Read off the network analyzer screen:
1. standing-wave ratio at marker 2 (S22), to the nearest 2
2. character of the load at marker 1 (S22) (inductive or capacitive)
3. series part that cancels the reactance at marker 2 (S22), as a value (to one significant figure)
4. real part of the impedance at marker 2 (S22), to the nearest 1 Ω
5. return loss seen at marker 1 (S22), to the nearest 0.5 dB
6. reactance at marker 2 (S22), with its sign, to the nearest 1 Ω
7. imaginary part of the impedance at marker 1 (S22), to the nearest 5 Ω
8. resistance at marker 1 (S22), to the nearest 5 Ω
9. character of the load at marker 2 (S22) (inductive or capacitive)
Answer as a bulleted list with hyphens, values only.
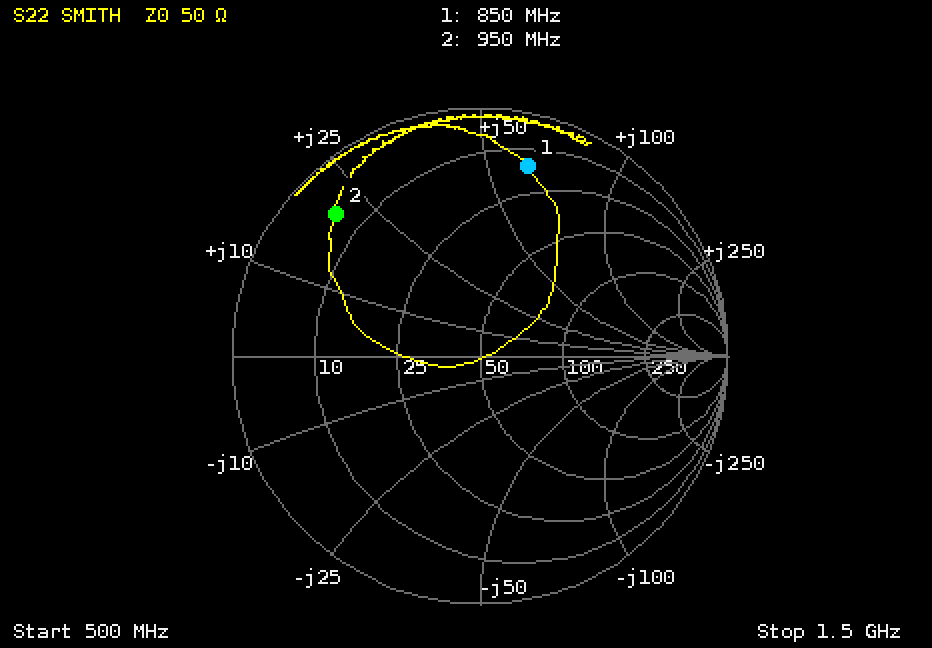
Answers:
- 10
- inductive
- 8 pF
- 6 Ω
- 2.0 dB
- +20 Ω
- +60 Ω
- 15 Ω
- inductive
